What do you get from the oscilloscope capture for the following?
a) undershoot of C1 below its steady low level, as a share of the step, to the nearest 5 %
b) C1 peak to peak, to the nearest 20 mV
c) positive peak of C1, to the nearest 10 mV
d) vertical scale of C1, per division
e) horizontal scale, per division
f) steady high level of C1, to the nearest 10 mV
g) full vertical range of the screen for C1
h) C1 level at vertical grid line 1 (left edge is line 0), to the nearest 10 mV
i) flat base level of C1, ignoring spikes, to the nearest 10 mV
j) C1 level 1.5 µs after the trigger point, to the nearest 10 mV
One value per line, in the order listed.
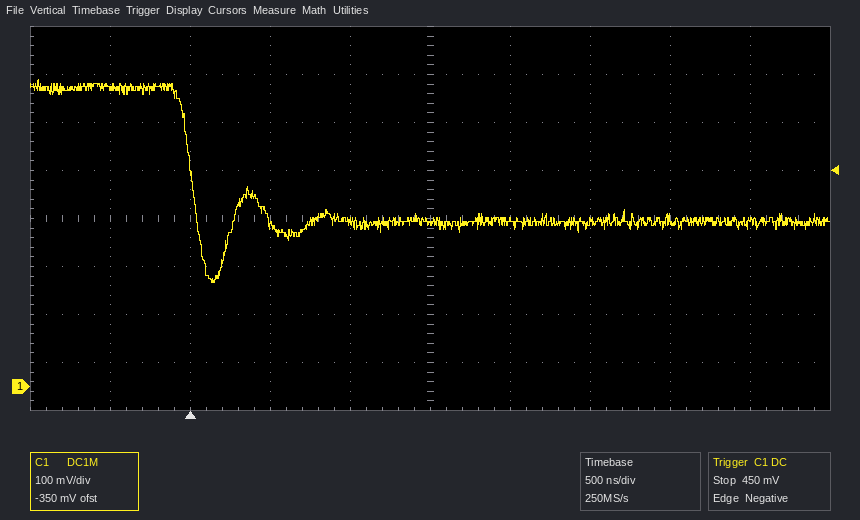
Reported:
45 %
420 mV
640 mV
100 mV
500 ns
620 mV
800 mV
620 mV
340 mV
340 mV
